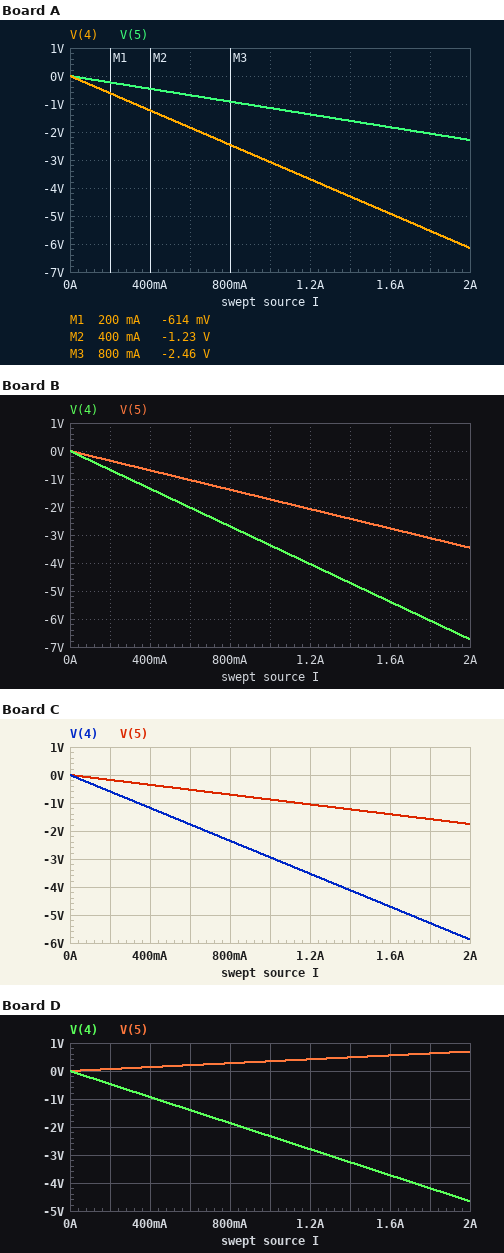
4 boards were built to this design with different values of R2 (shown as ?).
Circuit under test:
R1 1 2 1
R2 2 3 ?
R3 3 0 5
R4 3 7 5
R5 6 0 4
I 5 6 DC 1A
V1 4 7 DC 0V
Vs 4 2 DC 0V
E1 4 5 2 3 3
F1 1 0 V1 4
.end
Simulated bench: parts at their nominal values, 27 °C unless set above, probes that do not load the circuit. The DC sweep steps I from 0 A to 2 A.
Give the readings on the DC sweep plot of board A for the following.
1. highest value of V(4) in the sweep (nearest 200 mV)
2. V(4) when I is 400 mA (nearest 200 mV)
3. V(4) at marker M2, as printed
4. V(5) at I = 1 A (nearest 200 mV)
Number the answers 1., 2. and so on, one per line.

1. 0 V
2. -1.2 V
3. -1.23 V
4. -1.2 V
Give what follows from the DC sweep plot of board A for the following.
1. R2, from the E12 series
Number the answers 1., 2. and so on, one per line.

1. 1.8 Ω
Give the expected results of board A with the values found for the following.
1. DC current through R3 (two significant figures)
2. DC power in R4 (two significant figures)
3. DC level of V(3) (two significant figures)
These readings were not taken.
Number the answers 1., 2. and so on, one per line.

1. 490 mA
2. 83 mW
3. -2.4 V
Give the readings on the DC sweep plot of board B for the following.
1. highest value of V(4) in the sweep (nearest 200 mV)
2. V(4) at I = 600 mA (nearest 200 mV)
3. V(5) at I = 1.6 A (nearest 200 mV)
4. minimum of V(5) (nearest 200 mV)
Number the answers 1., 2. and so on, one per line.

1. 0 V
2. -2.0 V
3. -2.8 V
4. -3.4 V
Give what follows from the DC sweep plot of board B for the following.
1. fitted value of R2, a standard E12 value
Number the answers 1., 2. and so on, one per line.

1. 1.2 Ω
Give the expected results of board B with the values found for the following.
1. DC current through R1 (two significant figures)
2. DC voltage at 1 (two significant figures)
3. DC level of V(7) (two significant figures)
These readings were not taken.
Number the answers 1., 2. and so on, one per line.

1. 440 mA
2. -2.9 V
3. -3.4 V
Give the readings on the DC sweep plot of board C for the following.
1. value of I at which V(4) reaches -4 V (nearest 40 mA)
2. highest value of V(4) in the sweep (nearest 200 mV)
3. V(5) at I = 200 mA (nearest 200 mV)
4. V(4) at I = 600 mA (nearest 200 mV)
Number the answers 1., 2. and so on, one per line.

1. 1.36 A
2. 0 V
3. -200 mV
4. -1.8 V
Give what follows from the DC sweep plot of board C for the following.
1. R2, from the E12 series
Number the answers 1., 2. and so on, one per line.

1. 2.2 Ω
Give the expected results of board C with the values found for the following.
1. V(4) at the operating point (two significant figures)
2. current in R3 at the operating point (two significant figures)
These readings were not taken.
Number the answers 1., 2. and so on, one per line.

1. -2.9 V
2. 450 mA
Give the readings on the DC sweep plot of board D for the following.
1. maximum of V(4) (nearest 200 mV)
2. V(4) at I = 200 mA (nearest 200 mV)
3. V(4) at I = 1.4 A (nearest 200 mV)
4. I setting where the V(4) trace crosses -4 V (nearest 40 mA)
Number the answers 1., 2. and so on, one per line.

1. 0 V
2. -400 mV
3. -3.2 V
4. 1.72 A
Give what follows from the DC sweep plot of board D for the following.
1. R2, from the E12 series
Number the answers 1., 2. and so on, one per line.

1. 8.2 Ω
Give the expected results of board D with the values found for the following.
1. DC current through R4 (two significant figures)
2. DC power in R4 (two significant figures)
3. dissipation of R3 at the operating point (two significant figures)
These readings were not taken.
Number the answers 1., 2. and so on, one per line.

1. 180 mA
2. 160 mW
3. 410 mW
